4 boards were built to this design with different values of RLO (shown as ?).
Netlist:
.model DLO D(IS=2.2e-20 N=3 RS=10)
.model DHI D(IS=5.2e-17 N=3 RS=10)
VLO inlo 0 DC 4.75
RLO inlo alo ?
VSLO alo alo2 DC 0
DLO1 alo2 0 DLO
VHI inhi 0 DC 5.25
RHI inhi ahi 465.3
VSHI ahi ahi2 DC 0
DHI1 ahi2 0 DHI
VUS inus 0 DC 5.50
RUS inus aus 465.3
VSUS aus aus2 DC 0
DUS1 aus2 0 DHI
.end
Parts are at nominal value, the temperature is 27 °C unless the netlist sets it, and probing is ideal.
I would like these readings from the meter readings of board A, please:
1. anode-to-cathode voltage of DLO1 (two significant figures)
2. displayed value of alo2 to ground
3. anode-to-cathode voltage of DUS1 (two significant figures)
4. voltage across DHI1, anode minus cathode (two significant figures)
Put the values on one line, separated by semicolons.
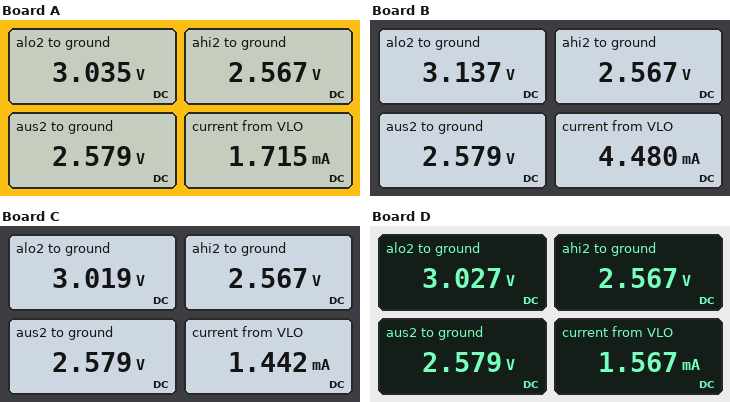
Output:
3.0 V; 3.035 V; 2.6 V; 2.6 V
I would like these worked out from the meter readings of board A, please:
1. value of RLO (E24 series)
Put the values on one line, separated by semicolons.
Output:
1 kΩ
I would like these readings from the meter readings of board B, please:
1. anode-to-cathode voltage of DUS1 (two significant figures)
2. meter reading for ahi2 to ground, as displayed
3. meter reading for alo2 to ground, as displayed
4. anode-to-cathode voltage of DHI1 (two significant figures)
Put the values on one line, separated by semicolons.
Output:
2.6 V; 2.567 V; 3.137 V; 2.6 V
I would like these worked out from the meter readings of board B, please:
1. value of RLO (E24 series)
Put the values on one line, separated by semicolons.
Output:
360 Ω
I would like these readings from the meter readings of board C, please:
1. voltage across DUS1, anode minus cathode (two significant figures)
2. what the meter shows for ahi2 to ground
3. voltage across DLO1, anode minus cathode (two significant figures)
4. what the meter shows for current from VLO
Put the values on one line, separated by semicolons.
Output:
2.6 V; 2.567 V; 3.0 V; 1.442 mA
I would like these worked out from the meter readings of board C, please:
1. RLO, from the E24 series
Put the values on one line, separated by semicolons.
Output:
1.2 kΩ
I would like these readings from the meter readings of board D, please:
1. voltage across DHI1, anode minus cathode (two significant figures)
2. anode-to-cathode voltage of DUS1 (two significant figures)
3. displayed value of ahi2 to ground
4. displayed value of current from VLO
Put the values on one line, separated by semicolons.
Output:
2.6 V; 2.6 V; 2.567 V; 1.567 mA
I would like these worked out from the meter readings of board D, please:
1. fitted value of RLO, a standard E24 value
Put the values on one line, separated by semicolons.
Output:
1.1 kΩ
